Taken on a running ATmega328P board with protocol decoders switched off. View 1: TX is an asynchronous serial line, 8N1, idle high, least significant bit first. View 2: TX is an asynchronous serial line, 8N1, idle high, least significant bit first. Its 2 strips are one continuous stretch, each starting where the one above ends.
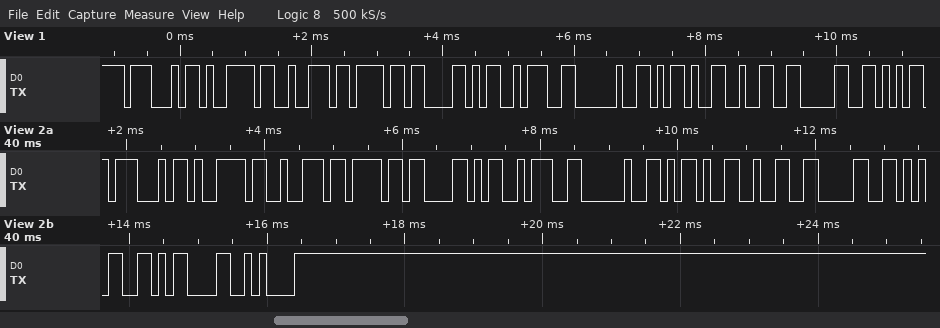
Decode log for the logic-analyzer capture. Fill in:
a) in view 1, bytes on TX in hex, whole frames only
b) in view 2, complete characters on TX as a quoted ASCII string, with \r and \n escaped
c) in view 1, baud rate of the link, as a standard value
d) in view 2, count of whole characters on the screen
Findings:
0x47 0x79 0x72 0x6F 0x58 0x3A 0x20 0x2D 0x32 0x30
"GyroX: -205\r\n"
9600 baud
13
